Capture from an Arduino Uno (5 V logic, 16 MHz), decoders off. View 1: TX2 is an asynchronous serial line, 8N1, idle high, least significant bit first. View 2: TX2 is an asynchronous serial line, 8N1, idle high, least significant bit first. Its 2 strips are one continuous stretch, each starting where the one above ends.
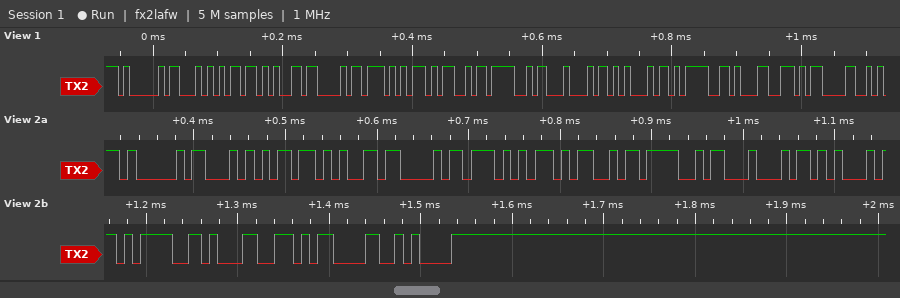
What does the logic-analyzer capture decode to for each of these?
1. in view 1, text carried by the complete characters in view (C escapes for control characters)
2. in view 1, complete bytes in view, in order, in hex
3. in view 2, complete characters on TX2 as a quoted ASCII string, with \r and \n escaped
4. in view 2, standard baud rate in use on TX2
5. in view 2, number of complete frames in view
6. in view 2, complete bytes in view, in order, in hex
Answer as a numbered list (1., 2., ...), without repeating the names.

1. "AT+CWMODE=1\r"
2. 41 54 2B 43 57 4D 4F 44 45 3D 31 0D
3. "AT+CWMODE=1\r\n"
4. 115200 baud
5. 13
6. 41 54 2B 43 57 4D 4F 44 45 3D 31 0D 0A
